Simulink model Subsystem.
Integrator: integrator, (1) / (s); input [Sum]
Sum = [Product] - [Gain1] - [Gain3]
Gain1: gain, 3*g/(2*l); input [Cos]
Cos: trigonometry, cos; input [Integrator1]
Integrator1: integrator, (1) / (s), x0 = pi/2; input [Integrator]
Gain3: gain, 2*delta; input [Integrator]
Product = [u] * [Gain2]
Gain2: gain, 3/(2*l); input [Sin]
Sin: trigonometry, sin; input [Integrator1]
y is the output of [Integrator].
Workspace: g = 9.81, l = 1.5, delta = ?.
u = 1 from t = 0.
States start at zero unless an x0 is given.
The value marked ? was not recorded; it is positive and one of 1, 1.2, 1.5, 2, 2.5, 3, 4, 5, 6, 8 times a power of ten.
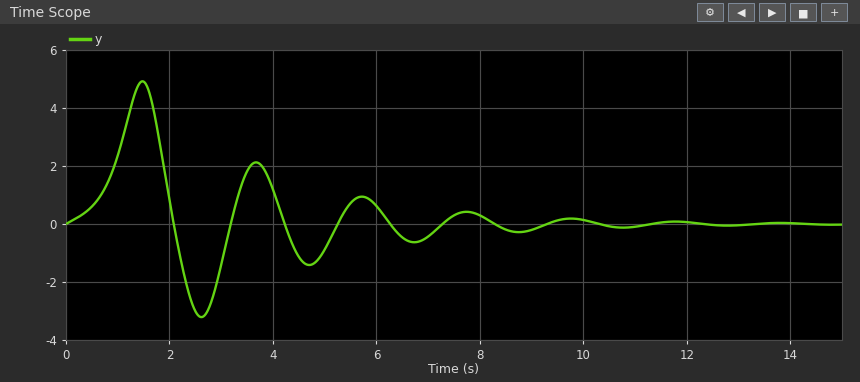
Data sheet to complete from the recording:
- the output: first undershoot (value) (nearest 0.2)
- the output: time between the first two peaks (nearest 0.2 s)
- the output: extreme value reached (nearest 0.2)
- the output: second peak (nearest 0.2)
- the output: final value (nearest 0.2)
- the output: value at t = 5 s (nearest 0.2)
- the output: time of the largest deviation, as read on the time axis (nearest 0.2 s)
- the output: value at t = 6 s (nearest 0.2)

-3.2
2.2 s
5.0
2.2
0.0
-0.8
1.4 s
0.6
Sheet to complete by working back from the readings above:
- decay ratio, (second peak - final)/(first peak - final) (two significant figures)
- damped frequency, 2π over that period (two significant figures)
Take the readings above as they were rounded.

0.44
2.9 rad/s
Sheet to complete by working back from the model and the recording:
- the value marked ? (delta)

0.4
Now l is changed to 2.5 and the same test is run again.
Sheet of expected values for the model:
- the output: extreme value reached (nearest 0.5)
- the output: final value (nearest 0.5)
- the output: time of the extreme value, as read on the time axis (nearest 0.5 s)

3.5
0.0
2.0 s
